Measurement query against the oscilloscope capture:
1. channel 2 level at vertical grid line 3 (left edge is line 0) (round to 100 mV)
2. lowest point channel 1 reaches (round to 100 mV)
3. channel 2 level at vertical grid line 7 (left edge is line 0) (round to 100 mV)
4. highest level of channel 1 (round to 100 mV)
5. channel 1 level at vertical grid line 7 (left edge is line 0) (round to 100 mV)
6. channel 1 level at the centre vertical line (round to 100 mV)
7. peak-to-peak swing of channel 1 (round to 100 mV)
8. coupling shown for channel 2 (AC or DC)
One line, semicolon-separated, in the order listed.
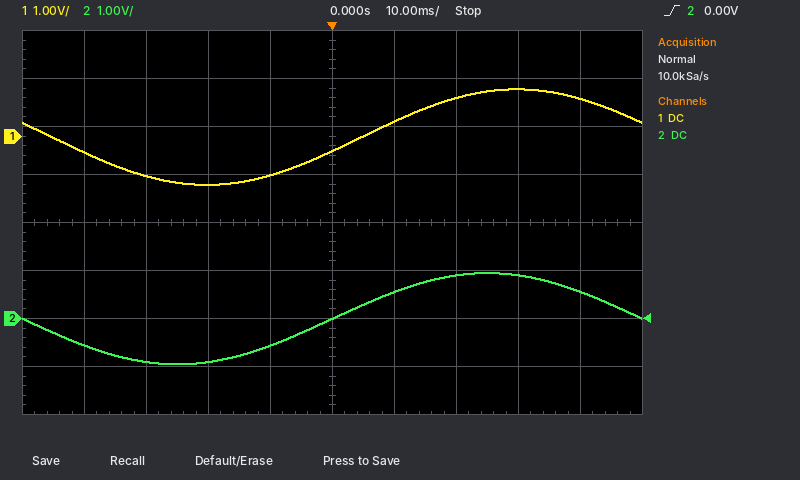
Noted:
-900 mV; -1.0 V; 900 mV; 1.0 V; 800 mV; -300 mV; 2.0 V; DC
